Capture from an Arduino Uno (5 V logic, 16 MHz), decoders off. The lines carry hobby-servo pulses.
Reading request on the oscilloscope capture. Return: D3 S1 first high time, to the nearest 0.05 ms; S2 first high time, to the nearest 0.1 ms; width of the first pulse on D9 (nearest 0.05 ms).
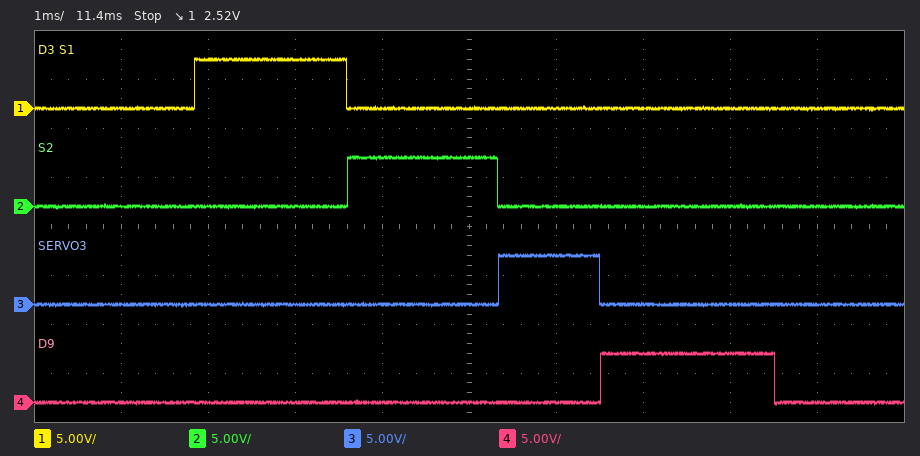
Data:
1.75 ms
1.7 ms
2.00 ms
